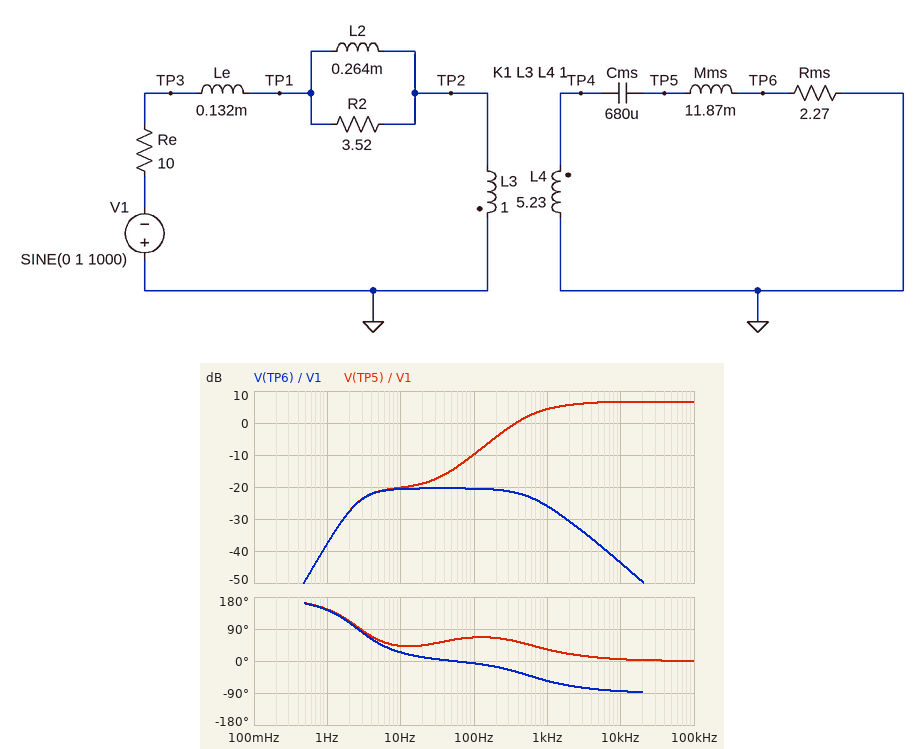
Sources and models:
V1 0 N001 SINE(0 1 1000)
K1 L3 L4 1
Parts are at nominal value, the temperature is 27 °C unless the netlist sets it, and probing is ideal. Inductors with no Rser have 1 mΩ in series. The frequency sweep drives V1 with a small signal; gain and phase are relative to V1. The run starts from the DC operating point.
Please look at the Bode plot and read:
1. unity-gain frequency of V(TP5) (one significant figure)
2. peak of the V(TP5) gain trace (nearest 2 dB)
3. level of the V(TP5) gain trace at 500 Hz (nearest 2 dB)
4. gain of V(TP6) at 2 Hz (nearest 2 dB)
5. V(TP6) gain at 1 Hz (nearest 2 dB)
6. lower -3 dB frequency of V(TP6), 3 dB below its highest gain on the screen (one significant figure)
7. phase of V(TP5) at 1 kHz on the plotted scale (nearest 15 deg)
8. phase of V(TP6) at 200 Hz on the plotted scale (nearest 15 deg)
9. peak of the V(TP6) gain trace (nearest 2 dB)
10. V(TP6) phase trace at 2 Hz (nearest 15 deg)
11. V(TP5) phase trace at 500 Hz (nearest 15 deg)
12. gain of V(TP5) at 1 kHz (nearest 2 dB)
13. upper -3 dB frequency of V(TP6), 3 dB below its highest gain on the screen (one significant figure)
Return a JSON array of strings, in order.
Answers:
["400 Hz", "6 dB", "2 dB", "-28 dB", "-38 dB", "3 Hz", "30 deg", "-15 deg", "-20 dB", "105 deg", "45 deg", "4 dB", "600 Hz"]
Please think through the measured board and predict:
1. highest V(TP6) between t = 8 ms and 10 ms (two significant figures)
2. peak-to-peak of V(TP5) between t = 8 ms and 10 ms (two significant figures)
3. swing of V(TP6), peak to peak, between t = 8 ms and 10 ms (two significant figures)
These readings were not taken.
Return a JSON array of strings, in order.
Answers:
["50 mV", "3.3 V", "100 mV"]
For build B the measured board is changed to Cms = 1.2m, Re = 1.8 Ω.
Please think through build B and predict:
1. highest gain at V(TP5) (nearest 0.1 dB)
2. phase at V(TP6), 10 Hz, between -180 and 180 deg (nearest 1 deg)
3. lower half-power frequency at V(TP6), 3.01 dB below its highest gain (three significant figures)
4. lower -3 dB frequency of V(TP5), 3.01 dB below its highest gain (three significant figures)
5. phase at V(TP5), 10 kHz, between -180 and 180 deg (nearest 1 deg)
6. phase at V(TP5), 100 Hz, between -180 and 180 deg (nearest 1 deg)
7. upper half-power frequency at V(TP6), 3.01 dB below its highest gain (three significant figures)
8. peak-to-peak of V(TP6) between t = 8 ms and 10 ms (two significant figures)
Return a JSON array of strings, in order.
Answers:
["6.7 dB", "48 deg", "10.3 Hz", "148 Hz", "2 deg", "41 deg", "143 Hz", "120 mV"]
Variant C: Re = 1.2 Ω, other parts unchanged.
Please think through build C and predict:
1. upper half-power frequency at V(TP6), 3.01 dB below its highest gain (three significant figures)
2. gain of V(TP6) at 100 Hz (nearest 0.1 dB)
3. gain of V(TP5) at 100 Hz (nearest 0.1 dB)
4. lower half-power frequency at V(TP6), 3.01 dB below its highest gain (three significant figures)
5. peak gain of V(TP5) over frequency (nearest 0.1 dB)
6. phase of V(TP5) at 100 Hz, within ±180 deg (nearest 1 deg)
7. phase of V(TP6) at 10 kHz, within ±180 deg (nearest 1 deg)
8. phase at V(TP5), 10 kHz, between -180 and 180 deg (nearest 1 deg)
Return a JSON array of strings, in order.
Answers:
["120 Hz", "-6.3 dB", "4.4 dB", "22.1 Hz", "6.7 dB", "36 deg", "-88 deg", "2 deg"]
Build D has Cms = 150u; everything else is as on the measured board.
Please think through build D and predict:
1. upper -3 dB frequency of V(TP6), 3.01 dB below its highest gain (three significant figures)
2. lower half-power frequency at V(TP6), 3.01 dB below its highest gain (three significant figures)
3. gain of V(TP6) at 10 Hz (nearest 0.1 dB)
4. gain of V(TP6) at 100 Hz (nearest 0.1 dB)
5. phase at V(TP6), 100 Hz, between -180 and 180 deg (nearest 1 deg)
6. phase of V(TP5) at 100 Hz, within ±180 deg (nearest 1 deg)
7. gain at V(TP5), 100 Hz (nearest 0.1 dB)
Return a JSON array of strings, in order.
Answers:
["629 Hz", "17.4 Hz", "-26.7 dB", "-20.4 dB", "2 deg", "75 deg", "-9.7 dB"]
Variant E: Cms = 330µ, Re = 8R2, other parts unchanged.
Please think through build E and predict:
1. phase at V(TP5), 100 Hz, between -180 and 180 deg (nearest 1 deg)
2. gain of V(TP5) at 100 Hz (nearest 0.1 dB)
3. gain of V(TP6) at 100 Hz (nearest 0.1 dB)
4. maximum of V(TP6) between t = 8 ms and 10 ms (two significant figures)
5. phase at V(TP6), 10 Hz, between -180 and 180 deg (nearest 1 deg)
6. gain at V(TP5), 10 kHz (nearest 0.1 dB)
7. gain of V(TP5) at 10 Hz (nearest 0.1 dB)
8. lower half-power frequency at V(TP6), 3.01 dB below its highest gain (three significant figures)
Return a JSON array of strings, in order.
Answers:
["68 deg", "-8.1 dB", "-18.8 dB", "52 mV", "51 deg", "6.6 dB", "-21.0 dB", "9.31 Hz"]
